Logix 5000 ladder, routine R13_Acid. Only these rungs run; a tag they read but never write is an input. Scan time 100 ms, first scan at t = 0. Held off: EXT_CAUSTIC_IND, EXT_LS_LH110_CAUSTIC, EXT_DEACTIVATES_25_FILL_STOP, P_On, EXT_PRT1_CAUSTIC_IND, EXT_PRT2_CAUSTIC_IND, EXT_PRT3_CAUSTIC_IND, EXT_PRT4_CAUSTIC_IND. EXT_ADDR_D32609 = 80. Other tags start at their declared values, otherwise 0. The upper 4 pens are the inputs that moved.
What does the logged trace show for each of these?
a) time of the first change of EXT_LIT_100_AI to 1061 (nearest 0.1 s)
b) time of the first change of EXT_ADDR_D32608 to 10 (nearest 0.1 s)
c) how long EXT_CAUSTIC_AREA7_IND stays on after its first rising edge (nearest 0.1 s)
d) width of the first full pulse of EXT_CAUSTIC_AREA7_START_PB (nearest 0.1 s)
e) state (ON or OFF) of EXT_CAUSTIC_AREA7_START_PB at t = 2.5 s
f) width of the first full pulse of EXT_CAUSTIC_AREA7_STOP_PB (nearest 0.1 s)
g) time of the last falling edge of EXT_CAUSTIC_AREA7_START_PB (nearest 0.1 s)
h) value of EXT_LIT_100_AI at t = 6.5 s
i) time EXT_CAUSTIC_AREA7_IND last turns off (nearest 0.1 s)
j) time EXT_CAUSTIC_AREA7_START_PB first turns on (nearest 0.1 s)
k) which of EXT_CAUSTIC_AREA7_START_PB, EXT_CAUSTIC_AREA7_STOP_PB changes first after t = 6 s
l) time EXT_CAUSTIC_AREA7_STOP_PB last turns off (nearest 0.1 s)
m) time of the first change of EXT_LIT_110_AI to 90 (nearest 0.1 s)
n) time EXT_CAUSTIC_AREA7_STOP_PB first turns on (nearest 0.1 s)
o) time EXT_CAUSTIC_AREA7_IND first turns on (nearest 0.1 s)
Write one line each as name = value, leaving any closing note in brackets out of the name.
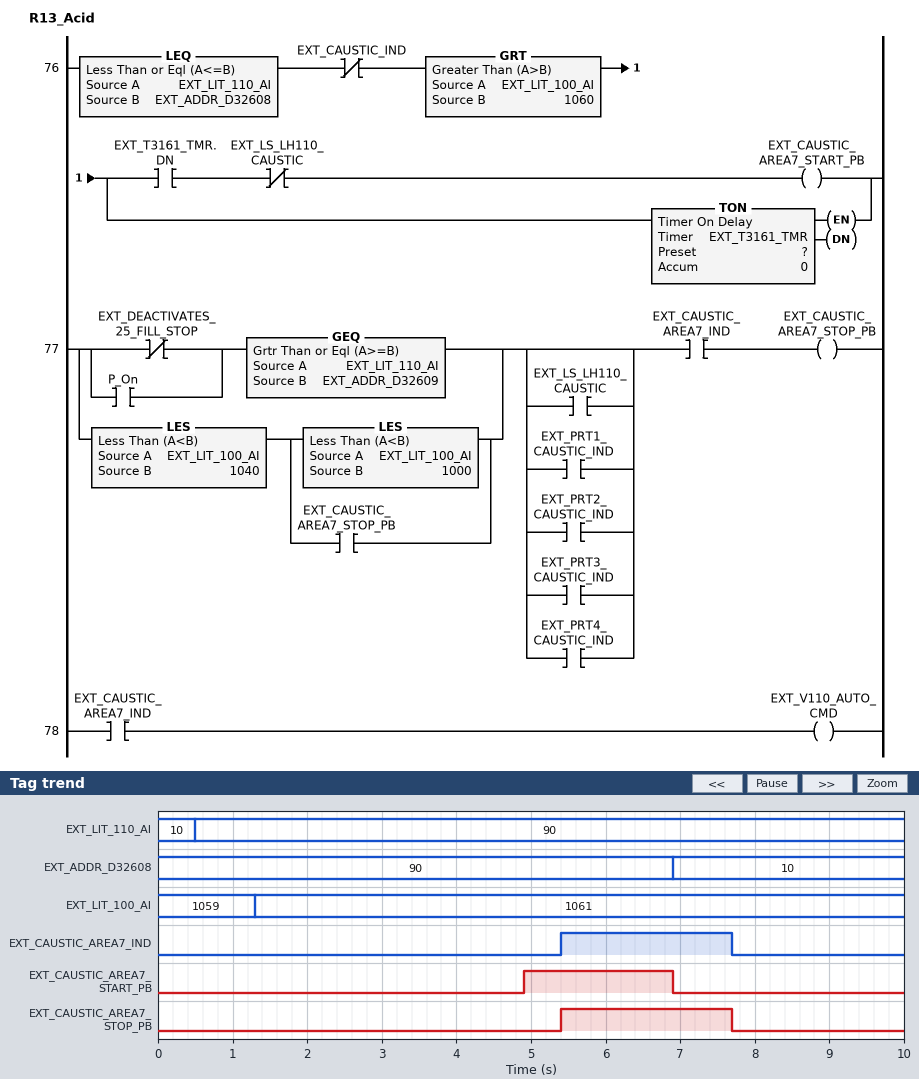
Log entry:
time of the first change of EXT_LIT_100_AI to 1061 = 1.3 s
time of the first change of EXT_ADDR_D32608 to 10 = 6.9 s
how long EXT_CAUSTIC_AREA7_IND stays on after its first rising edge = 2.3 s
width of the first full pulse of EXT_CAUSTIC_AREA7_START_PB = 2.0 s
state (ON or OFF) of EXT_CAUSTIC_AREA7_START_PB at t = 2.5 s = OFF
width of the first full pulse of EXT_CAUSTIC_AREA7_STOP_PB = 2.3 s
time of the last falling edge of EXT_CAUSTIC_AREA7_START_PB = 6.9 s
value of EXT_LIT_100_AI at t = 6.5 s = 1061
time EXT_CAUSTIC_AREA7_IND last turns off = 7.7 s
time EXT_CAUSTIC_AREA7_START_PB first turns on = 4.9 s
which of EXT_CAUSTIC_AREA7_START_PB, EXT_CAUSTIC_AREA7_STOP_PB changes first after t = 6 s = EXT_CAUSTIC_AREA7_START_PB
time EXT_CAUSTIC_AREA7_STOP_PB last turns off = 7.7 s
time of the first change of EXT_LIT_110_AI to 90 = 0.5 s
time EXT_CAUSTIC_AREA7_STOP_PB first turns on = 5.4 s
time EXT_CAUSTIC_AREA7_IND first turns on = 5.4 s
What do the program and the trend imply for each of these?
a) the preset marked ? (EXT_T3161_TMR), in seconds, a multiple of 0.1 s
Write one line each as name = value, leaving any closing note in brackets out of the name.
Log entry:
the preset marked ? (EXT_T3161_TMR), in seconds, a multiple of 0.1 s = 3.5 s
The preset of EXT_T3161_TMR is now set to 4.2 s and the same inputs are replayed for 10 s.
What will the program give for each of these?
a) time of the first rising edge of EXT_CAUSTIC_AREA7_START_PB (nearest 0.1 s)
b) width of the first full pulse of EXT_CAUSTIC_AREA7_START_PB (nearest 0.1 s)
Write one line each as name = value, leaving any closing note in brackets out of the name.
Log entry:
time of the first rising edge of EXT_CAUSTIC_AREA7_START_PB = 5.6 s
width of the first full pulse of EXT_CAUSTIC_AREA7_START_PB = 1.3 s
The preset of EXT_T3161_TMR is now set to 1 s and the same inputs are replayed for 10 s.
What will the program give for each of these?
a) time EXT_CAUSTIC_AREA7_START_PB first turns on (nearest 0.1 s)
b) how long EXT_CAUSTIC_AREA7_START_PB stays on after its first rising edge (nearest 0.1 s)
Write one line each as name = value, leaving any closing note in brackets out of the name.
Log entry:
time EXT_CAUSTIC_AREA7_START_PB first turns on = 2.4 s
how long EXT_CAUSTIC_AREA7_START_PB stays on after its first rising edge = 4.5 s
